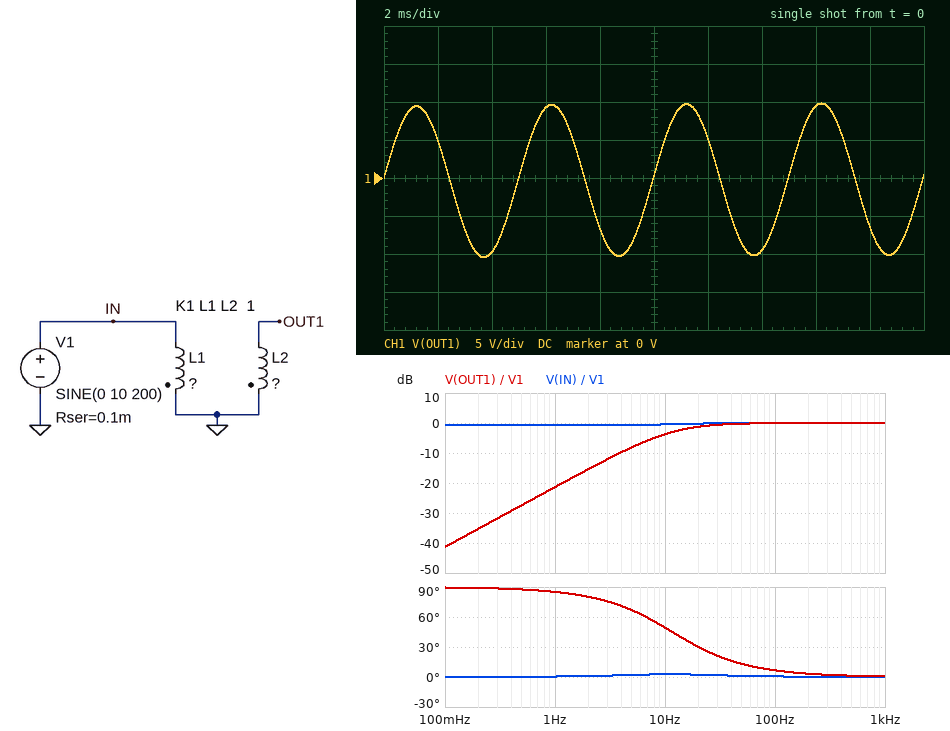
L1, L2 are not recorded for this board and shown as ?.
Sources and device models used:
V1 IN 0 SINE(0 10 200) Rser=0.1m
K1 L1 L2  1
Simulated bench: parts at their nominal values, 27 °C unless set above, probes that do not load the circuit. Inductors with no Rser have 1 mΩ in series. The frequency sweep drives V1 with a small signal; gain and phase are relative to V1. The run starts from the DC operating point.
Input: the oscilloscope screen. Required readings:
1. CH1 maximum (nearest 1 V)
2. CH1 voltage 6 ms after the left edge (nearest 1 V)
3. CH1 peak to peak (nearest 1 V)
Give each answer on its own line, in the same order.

10 V
9 V
20 V
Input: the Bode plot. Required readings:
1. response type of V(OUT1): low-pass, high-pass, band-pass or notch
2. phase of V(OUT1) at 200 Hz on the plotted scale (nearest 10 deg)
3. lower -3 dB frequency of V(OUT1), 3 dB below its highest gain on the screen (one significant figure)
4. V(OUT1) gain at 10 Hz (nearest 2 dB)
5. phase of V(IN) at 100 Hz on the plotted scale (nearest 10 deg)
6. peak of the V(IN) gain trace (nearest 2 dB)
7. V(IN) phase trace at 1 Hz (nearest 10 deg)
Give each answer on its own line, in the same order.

high-pass
0 deg
10 Hz
-4 dB
0 deg
0 dB
0 deg
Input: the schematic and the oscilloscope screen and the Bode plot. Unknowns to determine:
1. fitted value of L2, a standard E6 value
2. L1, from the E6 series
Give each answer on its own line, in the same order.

15 µH
15 µH
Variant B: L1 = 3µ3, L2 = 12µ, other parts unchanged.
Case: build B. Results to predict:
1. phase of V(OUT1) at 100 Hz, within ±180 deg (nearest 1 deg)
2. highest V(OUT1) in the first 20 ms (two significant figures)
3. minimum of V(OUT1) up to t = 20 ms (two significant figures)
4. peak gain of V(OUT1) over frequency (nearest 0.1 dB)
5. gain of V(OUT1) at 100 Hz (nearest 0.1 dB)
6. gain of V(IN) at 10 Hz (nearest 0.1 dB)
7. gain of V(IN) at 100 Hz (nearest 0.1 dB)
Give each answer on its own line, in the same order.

28 deg
18 V
-20 V
5.6 dB
4.5 dB
-0.8 dB
-0.2 dB
